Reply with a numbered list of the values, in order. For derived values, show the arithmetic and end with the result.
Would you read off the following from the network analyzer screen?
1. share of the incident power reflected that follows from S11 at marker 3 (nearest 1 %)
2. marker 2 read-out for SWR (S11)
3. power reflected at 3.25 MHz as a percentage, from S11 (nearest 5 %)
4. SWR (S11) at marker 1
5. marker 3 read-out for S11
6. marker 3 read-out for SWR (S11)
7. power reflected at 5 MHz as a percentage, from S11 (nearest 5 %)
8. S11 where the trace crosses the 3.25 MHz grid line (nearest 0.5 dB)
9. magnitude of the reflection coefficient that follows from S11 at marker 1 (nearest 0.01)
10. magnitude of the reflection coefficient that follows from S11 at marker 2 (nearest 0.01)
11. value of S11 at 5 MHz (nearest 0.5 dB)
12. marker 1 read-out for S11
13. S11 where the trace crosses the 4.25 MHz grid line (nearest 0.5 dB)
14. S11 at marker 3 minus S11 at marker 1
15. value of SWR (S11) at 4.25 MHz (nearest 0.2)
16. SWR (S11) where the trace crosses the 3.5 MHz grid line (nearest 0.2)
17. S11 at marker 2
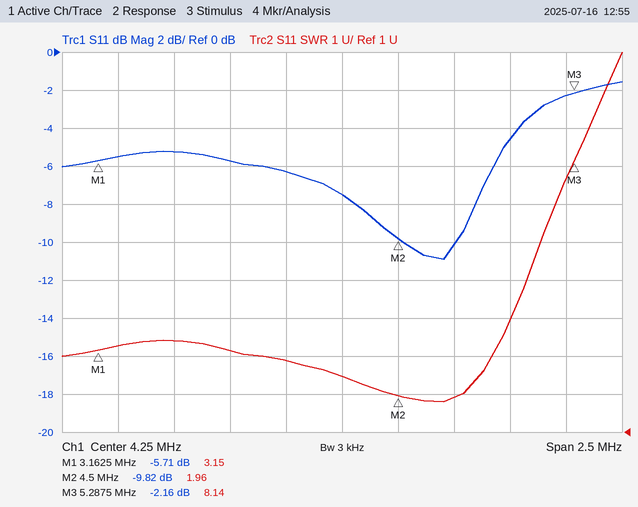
1. 10^(-2.16/10) ≈ 61 %
2. 1.96
3. 10^(-5.5/10) ≈ 28.2 %, so 30 % to the nearest 5 %
4. 3.15
5. -2.16 dB
6. 8.14
7. 10^(-4.5/10) ≈ 35 %
8. -5.5 dB
9. 10^(-5.71/20) ≈ 0.52
10. 10^(-9.82/20) ≈ 0.32
11. -4.5 dB
12. -5.71 dB
13. -7.5 dB
14. -2.16 − (-5.71) = 3.55 dB
15. 2.4
16. 3.4
17. -9.82 dB
